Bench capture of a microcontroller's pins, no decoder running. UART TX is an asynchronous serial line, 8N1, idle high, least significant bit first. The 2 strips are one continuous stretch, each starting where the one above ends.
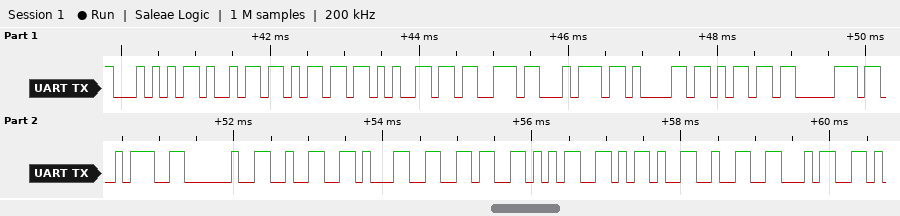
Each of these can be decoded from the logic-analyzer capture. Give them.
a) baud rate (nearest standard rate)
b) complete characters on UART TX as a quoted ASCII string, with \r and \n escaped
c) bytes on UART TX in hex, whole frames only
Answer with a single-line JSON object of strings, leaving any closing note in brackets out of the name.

{"baud rate": "9600 baud", "complete characters on UART TX as a quoted ASCII string, with \\r and \\n escaped": "\"Timestamp: 2165-24\"", "bytes on UART TX in hex, whole frames only": "54 69 6D 65 73 74 61 6D 70 3A 20 32 31 36 35 2D 32 34"}
